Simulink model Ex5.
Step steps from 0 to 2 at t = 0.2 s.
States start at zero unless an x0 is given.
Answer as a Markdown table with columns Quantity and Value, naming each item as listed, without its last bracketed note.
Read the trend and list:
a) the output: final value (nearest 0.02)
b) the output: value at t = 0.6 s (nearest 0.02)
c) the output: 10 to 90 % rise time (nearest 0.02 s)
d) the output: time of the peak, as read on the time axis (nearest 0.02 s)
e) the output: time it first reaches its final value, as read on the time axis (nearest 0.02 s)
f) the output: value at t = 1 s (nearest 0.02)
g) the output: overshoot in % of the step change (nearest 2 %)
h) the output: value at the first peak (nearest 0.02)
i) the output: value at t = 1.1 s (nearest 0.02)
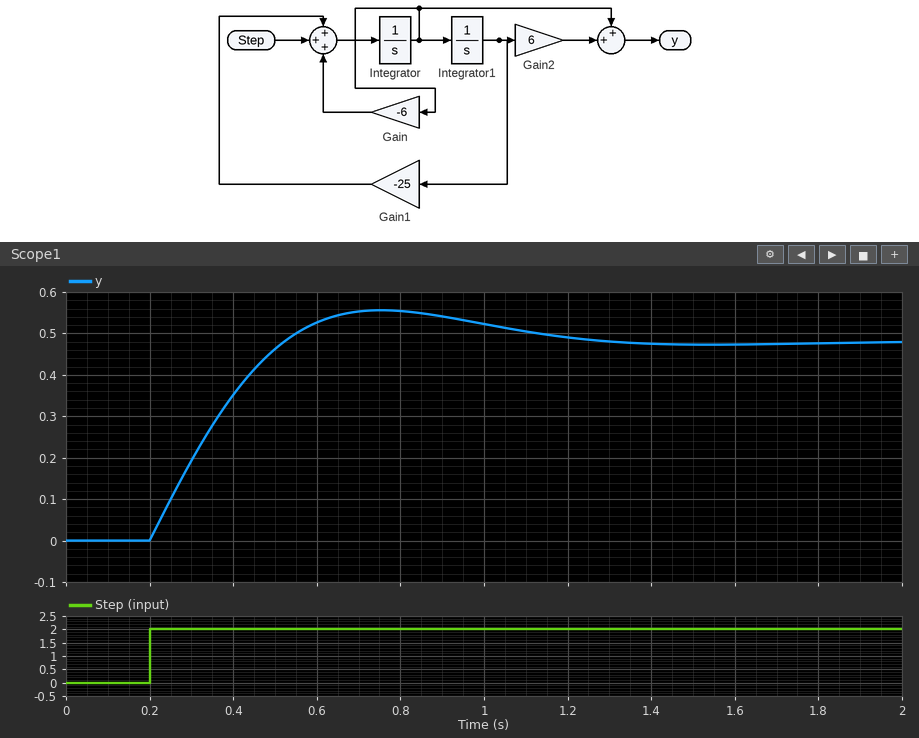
| Quantity | Value |
|---|---|
| the output: final value | 0.48 |
| the output: value at t = 0.6 s | 0.52 |
| the output: 10 to 90 % rise time | 0.24 s |
| the output: time of the peak, as read on the time axis | 0.76 s |
| the output: time it first reaches its final value, as read on the time axis | 0.52 s |
| the output: value at t = 1 s | 0.52 |
| the output: overshoot in % of the step change | 16 % |
| the output: value at the first peak | 0.56 |
| the output: value at t = 1.1 s | 0.50 |
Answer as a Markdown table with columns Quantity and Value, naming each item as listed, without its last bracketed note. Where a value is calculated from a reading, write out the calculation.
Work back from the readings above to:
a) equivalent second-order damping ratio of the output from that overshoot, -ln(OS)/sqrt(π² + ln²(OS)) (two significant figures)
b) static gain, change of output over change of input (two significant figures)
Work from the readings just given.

| Quantity | Value |
|---|---|
| equivalent second-order damping ratio of the output from that overshoot, -ln(OS)/sqrt(π² + ln²(OS)) | ln(0.16) = -1.833; 1.833 / sqrt(9.870 + 3.358) = 0.50 |
| static gain, change of output over change of input | (0.48 - 0) / (2 - 0) = 0.24 |
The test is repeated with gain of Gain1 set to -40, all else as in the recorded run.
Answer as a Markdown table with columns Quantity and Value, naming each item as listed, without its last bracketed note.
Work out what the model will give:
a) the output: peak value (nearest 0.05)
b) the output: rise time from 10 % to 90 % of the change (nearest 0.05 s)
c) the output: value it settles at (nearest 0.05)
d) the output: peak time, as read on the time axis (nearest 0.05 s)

| Quantity | Value |
|---|---|
| the output: peak value | 0.40 |
| the output: rise time from 10 % to 90 % of the change | 0.15 s |
| the output: value it settles at | 0.30 |
| the output: peak time, as read on the time axis | 0.55 s |
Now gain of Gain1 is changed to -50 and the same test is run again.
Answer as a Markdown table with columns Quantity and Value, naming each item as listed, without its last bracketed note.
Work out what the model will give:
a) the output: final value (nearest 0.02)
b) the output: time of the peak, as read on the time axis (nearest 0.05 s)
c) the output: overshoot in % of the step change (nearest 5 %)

| Quantity | Value |
|---|---|
| the output: final value | 0.24 |
| the output: time of the peak, as read on the time axis | 0.50 s |
| the output: overshoot in % of the step change | 45 % |
